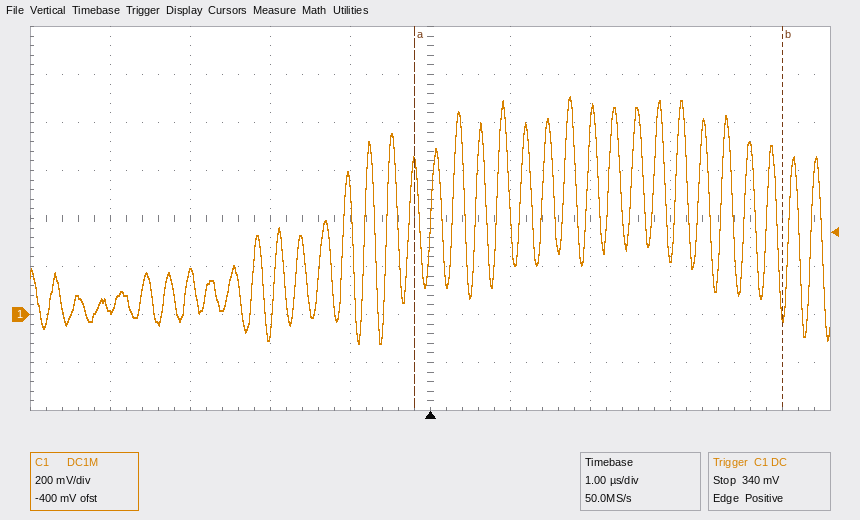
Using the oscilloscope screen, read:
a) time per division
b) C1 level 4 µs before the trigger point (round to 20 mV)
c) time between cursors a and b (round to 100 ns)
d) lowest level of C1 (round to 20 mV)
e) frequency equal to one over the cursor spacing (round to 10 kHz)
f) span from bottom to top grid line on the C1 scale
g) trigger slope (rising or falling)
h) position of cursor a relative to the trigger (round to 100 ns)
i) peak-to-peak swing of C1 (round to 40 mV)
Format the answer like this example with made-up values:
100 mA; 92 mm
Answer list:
1 µs; 20 mV; 4.6 µs; -120 mV; 220 kHz; 1.6 V; rising; -200 ns; 1.04 V
